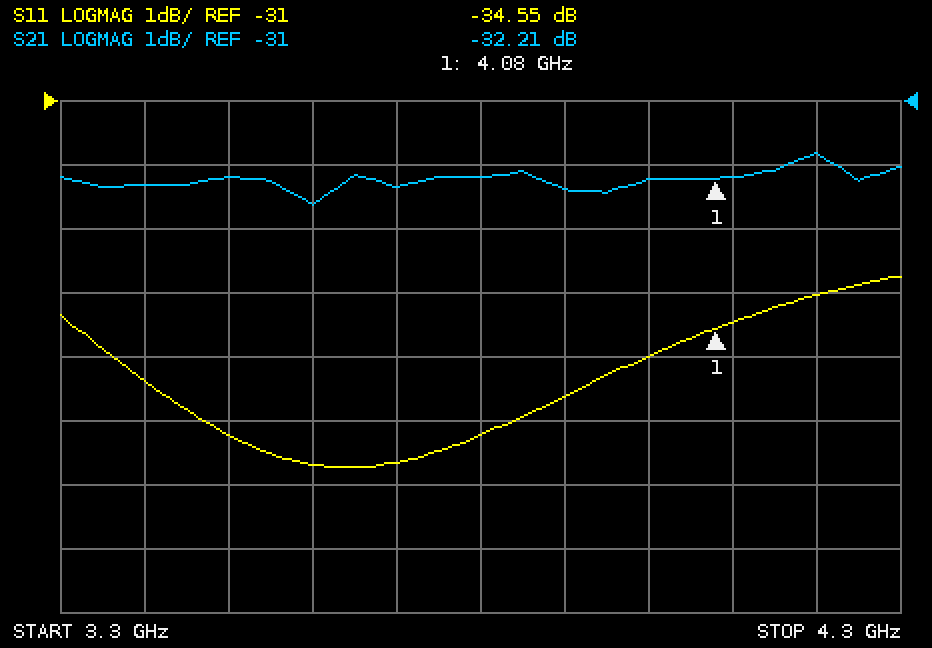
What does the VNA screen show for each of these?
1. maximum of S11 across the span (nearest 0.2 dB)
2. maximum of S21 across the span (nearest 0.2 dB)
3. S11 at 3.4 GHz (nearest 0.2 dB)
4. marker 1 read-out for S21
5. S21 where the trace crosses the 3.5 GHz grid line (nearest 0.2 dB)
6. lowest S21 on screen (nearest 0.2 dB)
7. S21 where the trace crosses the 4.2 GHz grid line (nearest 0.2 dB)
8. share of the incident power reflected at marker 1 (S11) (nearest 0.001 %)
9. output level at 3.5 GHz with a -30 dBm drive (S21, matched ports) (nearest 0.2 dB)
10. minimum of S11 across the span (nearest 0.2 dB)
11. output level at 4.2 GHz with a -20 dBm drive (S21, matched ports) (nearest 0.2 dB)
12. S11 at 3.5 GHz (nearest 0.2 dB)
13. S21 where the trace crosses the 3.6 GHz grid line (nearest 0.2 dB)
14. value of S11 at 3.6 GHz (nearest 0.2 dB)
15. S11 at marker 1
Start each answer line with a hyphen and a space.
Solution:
- -33.8 dB
- -31.8 dB
- -35.4 dB
- -32.21 dB
- -32.2 dB
- -32.6 dB
- -31.8 dB
- 0.035 %
- -62.2 dBm
- -36.8 dB
- -51.8 dBm
- -36.2 dB
- -32.6 dB
- -36.6 dB
- -34.55 dB
